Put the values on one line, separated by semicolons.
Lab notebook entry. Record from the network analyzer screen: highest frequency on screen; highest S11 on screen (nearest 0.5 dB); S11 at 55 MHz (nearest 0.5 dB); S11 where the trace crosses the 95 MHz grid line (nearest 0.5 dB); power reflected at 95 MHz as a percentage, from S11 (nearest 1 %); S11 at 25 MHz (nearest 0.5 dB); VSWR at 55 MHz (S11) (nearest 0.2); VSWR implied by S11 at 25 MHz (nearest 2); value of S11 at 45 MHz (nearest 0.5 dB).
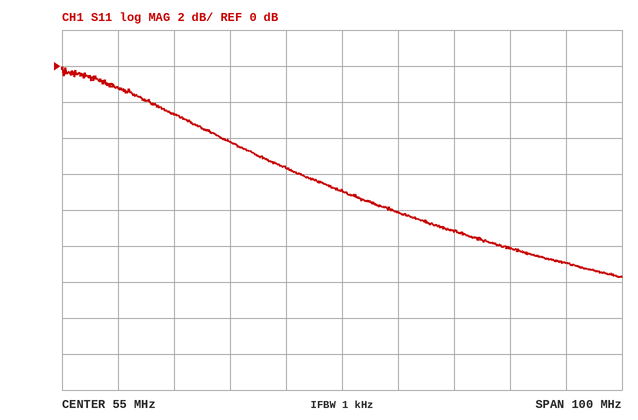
105 MHz; 0.0 dB; -7.0 dB; -11.0 dB; 8 %; -2.5 dB; 2.6; 6; -5.5 dB
